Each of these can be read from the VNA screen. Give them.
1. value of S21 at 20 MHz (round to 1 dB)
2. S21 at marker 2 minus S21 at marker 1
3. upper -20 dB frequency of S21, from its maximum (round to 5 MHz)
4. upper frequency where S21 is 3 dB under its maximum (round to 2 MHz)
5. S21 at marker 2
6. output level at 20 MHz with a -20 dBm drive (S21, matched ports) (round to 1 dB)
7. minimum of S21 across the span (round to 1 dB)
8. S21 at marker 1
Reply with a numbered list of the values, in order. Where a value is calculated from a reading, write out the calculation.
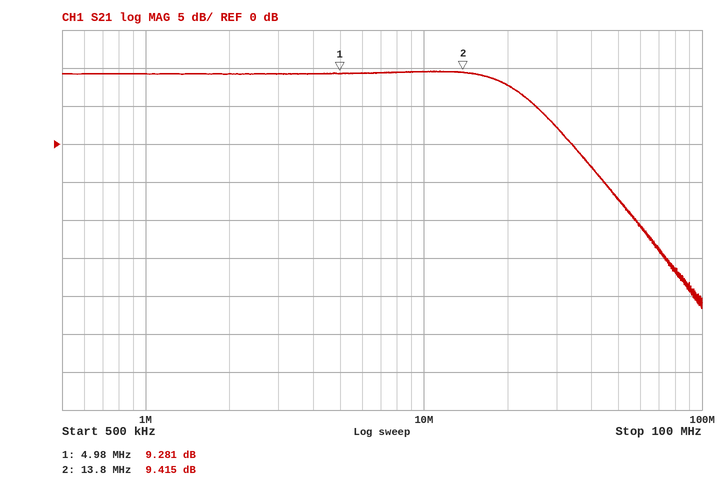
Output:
1. 8 dB
2. 9.415 − (9.281) = 0.134 dB
3. 60 MHz
4. 22 MHz
5. 9.415 dB
6. -20 dBm + (8 dB) = -12 dBm
7. -22 dB
8. 9.281 dB
